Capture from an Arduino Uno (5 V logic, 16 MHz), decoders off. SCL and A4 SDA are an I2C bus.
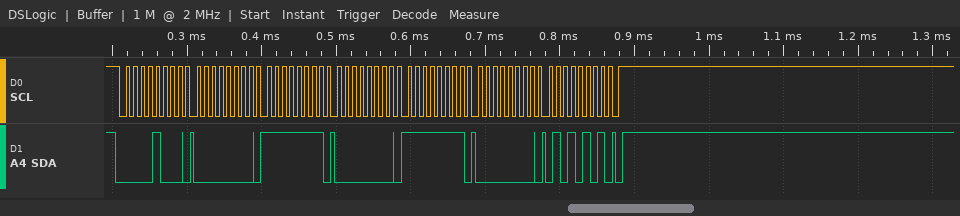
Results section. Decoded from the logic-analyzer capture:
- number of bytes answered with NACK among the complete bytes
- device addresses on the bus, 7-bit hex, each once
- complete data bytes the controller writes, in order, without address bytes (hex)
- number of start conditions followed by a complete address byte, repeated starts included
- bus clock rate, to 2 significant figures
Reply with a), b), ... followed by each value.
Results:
a) 0
b) 0x04
c) 00 FF 00 FF 00 55
d) 1
e) 100 kHz
